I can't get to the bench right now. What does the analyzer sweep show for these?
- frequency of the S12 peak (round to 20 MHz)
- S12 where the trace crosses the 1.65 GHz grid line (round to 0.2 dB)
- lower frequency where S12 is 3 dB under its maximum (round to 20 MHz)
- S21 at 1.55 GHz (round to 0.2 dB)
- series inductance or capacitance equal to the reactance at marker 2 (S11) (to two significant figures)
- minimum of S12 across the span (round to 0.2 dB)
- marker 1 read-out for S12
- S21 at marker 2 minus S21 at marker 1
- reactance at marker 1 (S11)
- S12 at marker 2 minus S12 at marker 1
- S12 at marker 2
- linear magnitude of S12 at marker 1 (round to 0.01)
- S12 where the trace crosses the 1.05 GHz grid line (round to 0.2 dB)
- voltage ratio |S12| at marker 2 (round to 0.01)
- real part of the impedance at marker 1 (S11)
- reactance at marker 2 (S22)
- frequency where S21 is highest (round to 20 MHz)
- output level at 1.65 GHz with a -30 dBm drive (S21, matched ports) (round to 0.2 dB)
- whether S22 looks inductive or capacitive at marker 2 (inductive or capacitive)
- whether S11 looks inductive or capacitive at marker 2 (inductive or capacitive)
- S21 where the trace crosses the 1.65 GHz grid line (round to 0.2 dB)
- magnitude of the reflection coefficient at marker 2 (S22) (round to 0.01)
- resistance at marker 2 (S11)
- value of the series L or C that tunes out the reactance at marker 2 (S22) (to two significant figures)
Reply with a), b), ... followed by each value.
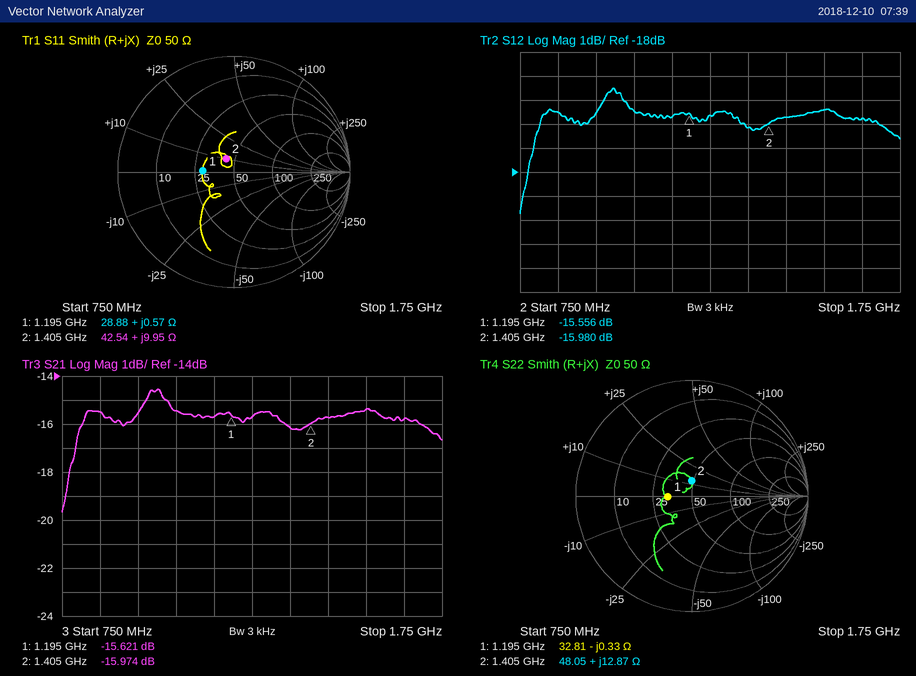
a) 1.00 GHz
b) -15.8 dB
c) 780 MHz
d) -15.4 dB
e) 1.1 nH
f) -19.8 dB
g) -15.556 dB
h) -0.353 dB
i) +0.57 Ω
j) -0.424 dB
k) -15.980 dB
l) 0.17
m) -15.4 dB
n) 0.16
o) 28.88 Ω
p) +12.87 Ω
q) 1.00 GHz
r) -45.8 dBm
s) inductive
t) inductive
u) -15.8 dB
v) 0.13
w) 42.54 Ω
x) 8.8 pF
